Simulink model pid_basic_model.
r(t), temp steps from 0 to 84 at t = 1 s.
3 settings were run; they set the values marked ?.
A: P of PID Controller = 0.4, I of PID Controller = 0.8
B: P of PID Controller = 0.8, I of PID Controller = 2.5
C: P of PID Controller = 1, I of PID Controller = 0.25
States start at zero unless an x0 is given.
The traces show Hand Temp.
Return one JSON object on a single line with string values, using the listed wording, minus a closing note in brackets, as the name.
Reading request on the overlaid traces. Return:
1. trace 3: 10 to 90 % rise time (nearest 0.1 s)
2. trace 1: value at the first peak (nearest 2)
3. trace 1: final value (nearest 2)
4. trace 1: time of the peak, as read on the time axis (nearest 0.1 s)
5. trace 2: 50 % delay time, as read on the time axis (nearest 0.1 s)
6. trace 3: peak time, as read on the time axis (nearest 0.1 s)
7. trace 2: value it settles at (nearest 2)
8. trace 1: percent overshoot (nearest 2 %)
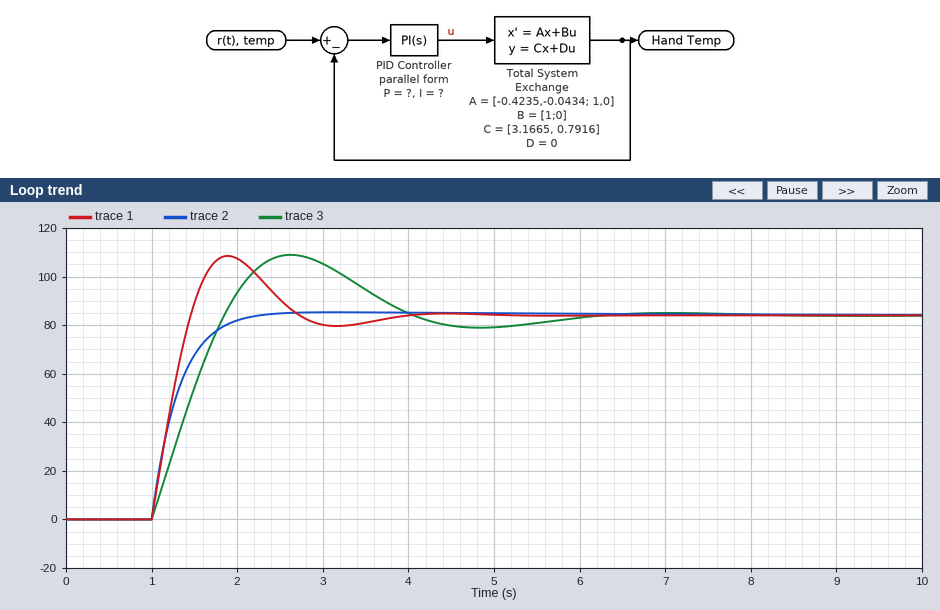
{"trace 3: 10 to 90 % rise time": "0.7 s", "trace 1: value at the first peak": "108", "trace 1: final value": "84", "trace 1: time of the peak, as read on the time axis": "1.9 s", "trace 2: 50 % delay time, as read on the time axis": "1.2 s", "trace 3: peak time, as read on the time axis": "2.6 s", "trace 2: value it settles at": "84", "trace 1: percent overshoot": "30 %"}
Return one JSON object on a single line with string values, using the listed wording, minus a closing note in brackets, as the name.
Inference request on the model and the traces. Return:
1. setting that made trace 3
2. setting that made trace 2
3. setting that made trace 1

{"setting that made trace 3": "A", "setting that made trace 2": "C", "setting that made trace 1": "B"}
